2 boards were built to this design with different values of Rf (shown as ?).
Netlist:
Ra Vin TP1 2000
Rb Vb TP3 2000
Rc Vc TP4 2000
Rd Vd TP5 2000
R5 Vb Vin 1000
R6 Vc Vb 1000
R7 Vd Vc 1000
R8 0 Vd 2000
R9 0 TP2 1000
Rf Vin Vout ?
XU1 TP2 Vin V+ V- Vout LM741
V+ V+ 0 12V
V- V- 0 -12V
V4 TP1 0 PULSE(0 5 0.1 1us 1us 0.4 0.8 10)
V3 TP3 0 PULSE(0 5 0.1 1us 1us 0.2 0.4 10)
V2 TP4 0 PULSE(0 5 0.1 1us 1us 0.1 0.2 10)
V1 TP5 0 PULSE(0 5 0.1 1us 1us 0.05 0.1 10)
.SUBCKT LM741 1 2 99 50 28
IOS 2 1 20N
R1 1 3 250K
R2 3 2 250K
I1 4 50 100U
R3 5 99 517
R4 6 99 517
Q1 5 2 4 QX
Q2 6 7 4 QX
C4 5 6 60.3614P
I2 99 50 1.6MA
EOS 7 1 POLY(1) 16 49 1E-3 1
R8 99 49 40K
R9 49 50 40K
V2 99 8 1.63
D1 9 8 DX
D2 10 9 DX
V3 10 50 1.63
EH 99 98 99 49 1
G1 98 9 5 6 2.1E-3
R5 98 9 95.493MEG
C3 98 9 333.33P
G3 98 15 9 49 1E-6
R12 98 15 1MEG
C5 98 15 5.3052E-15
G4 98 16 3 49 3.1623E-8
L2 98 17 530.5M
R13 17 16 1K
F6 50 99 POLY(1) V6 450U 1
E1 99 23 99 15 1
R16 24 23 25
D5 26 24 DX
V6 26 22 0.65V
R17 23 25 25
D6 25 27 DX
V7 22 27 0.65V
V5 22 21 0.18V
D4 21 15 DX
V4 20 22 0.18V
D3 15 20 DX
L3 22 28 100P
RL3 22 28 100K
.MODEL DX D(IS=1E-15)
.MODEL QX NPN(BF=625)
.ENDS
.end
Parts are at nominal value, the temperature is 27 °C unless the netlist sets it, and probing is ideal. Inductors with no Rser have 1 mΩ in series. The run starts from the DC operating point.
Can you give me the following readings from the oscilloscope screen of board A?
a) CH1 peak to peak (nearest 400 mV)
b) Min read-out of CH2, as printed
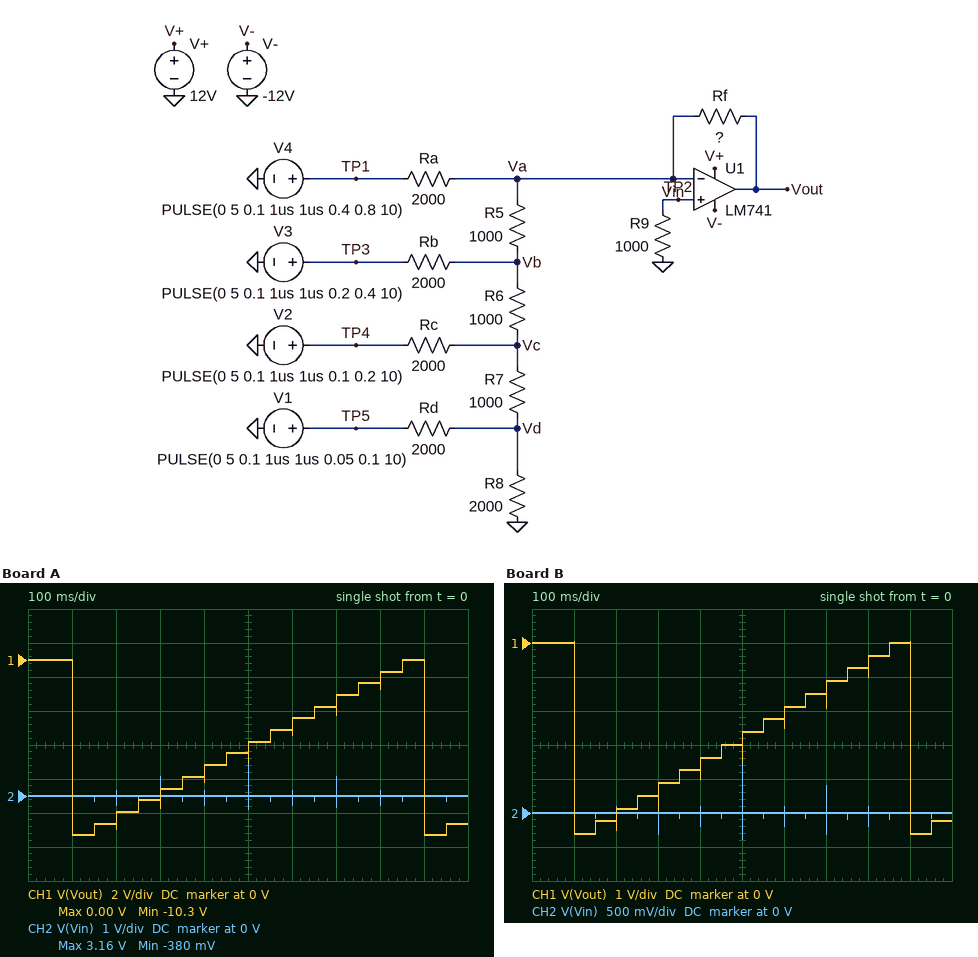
10.4 V
-380 mV
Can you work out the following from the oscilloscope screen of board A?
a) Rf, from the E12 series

2.2 kΩ
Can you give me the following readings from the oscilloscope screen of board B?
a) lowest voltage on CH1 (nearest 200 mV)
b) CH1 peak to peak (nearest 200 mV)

-5.6 V
5.6 V
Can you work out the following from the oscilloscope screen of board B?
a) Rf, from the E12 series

1.2 kΩ
